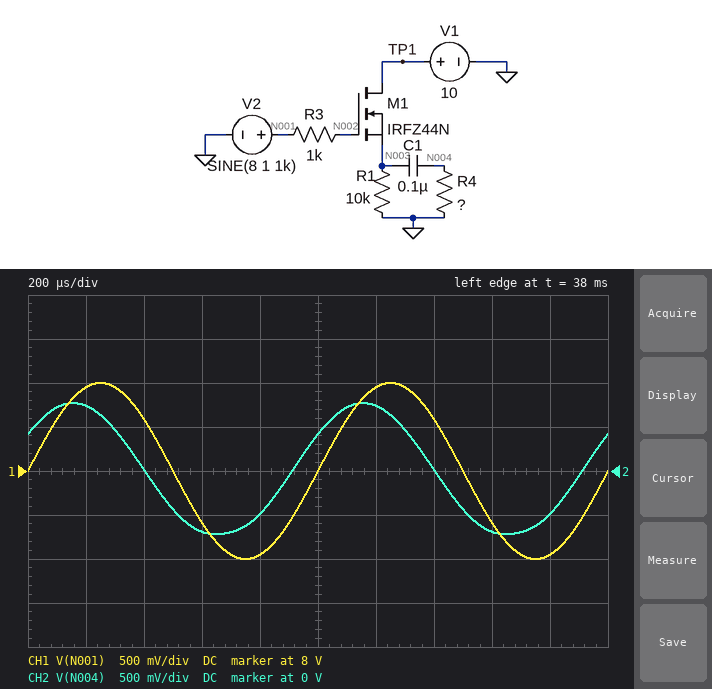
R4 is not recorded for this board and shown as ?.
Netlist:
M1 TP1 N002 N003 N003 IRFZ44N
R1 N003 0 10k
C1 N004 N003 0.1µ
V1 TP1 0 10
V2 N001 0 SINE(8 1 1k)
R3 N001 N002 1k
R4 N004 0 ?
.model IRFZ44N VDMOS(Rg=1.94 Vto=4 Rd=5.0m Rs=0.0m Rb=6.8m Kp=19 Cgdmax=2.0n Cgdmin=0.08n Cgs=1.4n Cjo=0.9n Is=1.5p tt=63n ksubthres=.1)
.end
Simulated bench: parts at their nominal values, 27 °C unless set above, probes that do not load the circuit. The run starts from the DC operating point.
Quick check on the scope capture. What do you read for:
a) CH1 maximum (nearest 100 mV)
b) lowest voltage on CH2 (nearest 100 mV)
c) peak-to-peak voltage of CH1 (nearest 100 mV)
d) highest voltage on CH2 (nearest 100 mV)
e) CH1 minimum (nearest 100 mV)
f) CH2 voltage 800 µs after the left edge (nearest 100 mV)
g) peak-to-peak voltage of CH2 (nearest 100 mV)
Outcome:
9.0 V
-700 mV
2.0 V
800 mV
7.0 V
-500 mV
1.5 V
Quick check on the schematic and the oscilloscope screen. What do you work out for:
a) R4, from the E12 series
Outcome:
2.2 kΩ
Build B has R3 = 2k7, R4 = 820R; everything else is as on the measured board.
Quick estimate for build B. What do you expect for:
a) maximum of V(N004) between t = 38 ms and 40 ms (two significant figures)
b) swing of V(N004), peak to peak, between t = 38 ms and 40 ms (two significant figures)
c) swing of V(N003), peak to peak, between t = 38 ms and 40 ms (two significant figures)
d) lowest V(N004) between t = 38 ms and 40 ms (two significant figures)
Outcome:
440 mV
780 mV
1.8 V
-340 mV
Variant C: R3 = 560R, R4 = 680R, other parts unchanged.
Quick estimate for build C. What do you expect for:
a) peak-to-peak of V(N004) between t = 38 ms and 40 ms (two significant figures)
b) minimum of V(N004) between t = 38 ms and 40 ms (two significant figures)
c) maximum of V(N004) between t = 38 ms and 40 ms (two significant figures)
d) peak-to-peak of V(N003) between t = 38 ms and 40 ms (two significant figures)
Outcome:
670 mV
-290 mV
380 mV
1.8 V
